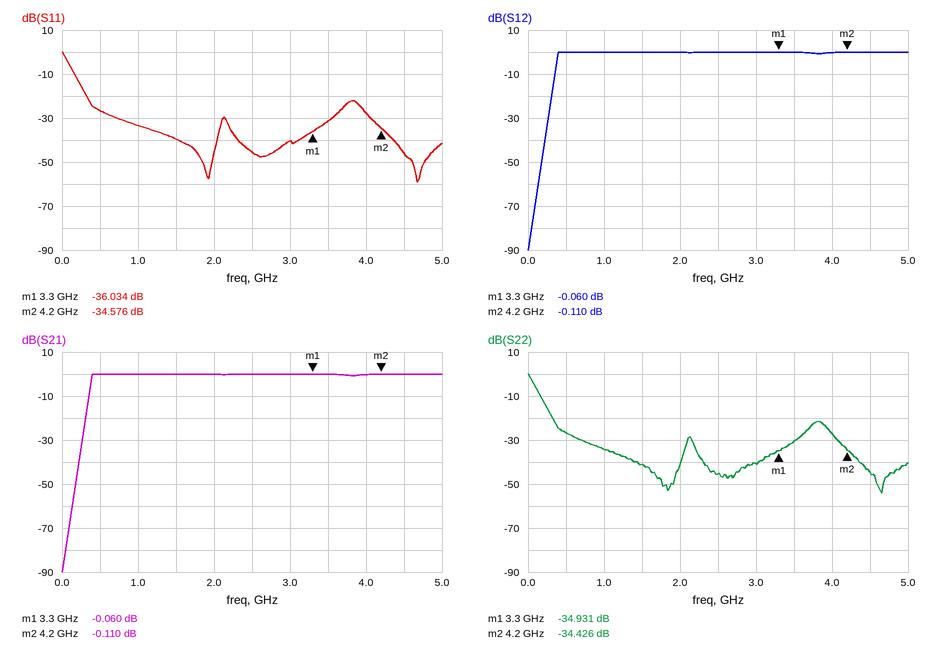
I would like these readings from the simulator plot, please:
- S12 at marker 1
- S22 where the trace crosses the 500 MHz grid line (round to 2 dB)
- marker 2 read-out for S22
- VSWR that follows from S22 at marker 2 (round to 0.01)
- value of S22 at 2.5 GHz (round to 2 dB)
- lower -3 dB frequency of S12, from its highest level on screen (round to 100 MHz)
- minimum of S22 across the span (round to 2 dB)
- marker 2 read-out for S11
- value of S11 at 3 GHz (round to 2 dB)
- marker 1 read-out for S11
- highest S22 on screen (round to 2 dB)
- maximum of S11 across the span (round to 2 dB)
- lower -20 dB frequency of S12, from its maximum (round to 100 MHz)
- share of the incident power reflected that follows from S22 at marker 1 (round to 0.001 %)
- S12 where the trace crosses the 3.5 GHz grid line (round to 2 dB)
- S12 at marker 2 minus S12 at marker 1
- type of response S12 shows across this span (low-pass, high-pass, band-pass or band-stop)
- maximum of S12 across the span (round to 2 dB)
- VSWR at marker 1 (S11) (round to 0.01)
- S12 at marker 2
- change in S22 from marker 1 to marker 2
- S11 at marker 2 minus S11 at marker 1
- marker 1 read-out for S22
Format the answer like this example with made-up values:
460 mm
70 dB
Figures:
-0.060 dB
-26 dB
-34.426 dB
1.04
-46 dB
400 MHz
-54 dB
-34.576 dB
-40 dB
-36.034 dB
0 dB
0 dB
300 MHz
0.032 %
0 dB
-0.050 dB
high-pass
0 dB
1.03
-0.110 dB
0.505 dB
1.458 dB
-34.931 dB
